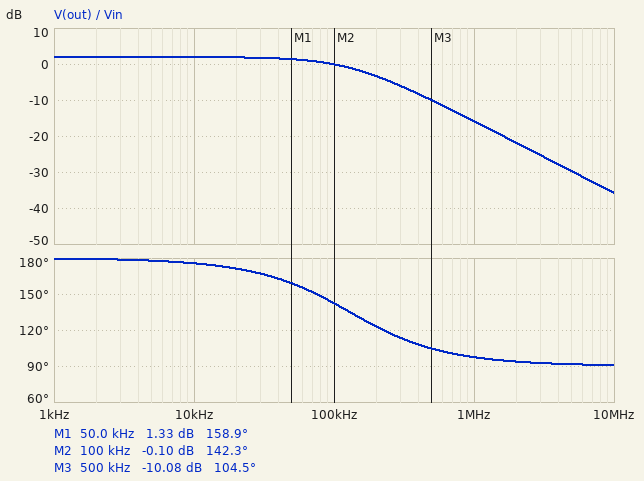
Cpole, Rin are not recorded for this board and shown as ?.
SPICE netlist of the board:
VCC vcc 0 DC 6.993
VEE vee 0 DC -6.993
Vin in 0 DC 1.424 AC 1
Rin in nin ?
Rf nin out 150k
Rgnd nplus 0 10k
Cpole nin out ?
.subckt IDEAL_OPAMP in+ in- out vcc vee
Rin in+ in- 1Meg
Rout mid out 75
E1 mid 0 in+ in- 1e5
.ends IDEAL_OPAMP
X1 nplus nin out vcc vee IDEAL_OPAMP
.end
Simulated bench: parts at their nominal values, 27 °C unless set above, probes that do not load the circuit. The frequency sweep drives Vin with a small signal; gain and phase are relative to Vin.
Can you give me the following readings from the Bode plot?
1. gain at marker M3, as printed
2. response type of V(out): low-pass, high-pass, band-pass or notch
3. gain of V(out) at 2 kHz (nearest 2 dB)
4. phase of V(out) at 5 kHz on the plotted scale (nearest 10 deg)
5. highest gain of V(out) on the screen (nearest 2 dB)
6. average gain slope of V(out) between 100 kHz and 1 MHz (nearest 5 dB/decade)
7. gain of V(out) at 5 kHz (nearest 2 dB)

-10.08 dB
low-pass
2 dB
180 deg
2 dB
-15 dB/decade
2 dB
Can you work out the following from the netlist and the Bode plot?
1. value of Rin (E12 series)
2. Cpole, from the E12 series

120 kΩ
8.2 pF
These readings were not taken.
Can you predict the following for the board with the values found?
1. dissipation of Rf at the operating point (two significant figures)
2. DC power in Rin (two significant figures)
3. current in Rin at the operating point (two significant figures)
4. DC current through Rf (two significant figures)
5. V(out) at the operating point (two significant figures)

21 µW
17 µW
12 µA
12 µA
-1.8 V
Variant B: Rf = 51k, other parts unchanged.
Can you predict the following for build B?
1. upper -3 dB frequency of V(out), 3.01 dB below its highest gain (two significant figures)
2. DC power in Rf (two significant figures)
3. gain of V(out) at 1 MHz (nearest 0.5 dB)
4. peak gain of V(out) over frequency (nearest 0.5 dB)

380 kHz
7.2 µW
-16.5 dB
-7.5 dB
